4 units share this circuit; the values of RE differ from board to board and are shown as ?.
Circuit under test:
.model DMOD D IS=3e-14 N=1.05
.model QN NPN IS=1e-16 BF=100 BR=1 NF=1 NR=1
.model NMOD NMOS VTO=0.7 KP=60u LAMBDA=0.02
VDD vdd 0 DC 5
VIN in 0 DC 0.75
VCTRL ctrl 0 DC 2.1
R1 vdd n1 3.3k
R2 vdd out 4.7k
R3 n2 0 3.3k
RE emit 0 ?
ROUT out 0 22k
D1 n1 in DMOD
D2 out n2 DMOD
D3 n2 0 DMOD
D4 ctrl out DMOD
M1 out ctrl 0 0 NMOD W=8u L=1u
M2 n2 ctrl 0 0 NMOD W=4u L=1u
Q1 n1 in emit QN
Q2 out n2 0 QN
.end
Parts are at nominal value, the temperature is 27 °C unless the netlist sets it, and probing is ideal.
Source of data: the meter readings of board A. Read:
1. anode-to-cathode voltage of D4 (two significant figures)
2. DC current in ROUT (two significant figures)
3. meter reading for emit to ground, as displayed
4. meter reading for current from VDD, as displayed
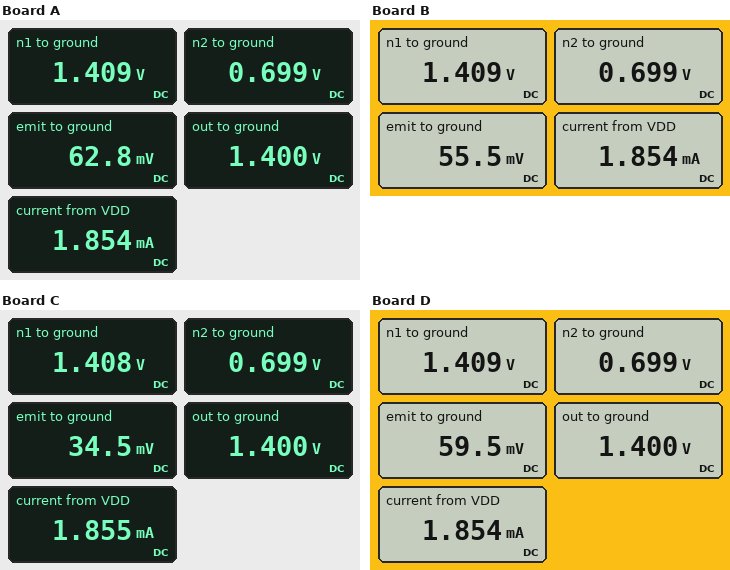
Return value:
700 mV
64 µA
62.8 mV
1.854 mA
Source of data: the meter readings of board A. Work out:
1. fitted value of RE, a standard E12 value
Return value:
1.8 kΩ
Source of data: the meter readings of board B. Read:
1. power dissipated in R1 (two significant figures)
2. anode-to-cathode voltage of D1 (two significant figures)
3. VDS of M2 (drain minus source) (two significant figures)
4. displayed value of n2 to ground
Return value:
3.9 mW
660 mV
700 mV
0.699 V
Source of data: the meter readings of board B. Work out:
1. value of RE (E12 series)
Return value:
1.2 kΩ
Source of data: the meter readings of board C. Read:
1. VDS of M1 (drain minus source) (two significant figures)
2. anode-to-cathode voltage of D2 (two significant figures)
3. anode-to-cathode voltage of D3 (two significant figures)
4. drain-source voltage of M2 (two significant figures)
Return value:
1.4 V
700 mV
700 mV
700 mV
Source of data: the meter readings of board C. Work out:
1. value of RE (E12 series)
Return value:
330 Ω
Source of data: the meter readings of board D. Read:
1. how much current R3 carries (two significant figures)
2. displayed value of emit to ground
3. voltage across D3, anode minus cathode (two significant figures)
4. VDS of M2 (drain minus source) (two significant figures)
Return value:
210 µA
59.5 mV
700 mV
700 mV
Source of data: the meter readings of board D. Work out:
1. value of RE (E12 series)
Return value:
1.5 kΩ
